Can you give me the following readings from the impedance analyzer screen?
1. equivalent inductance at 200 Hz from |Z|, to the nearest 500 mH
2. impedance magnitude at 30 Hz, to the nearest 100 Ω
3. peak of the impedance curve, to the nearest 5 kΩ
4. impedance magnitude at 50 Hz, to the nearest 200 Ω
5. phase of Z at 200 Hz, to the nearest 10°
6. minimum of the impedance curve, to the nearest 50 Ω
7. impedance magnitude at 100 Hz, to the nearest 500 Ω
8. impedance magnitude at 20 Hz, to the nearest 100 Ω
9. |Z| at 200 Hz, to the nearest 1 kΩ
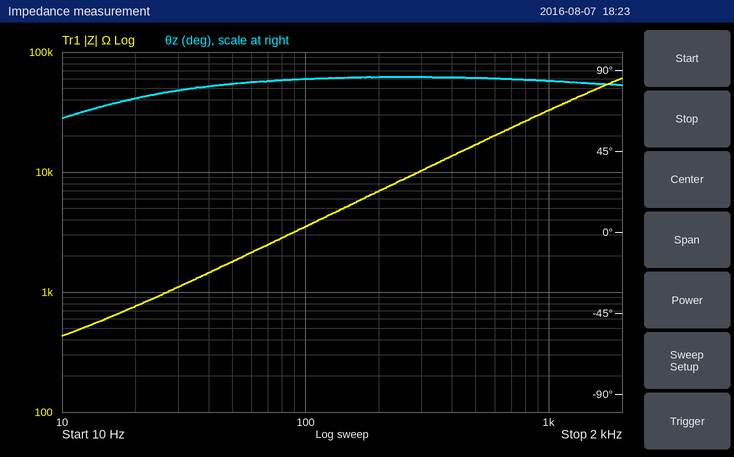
5.5 H
1.1 kΩ
60 kΩ
1.8 kΩ
90°
450 Ω
3.5 kΩ
800 Ω
7 kΩ
